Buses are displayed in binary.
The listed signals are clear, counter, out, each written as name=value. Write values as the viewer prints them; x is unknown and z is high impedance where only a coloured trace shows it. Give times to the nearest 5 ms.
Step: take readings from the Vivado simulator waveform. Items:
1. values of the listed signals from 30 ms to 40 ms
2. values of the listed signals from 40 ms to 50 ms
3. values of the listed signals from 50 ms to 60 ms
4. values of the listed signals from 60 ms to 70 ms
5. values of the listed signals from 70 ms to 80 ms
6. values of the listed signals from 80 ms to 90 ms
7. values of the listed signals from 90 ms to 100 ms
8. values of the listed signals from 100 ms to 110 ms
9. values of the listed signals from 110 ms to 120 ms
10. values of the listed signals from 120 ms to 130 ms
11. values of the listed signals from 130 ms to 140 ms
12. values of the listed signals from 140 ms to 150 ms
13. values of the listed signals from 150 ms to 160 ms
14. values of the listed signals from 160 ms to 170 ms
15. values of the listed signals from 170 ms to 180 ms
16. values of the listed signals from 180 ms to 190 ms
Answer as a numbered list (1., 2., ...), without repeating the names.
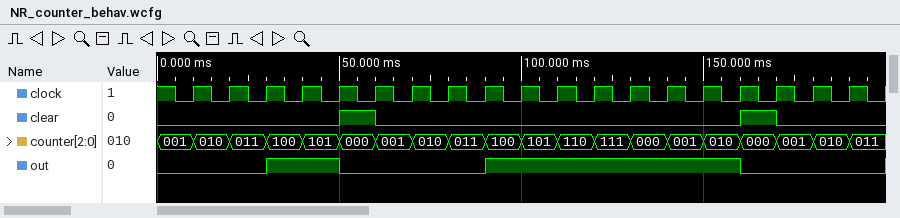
1. clear=0, counter=100, out=1
2. clear=0, counter=101, out=1
3. clear=1, counter=000, out=0
4. clear=0, counter=001, out=0
5. clear=0, counter=010, out=0
6. clear=0, counter=011, out=0
7. clear=0, counter=100, out=1
8. clear=0, counter=101, out=1
9. clear=0, counter=110, out=1
10. clear=0, counter=111, out=1
11. clear=0, counter=000, out=1
12. clear=0, counter=001, out=1
13. clear=0, counter=010, out=1
14. clear=1, counter=000, out=0
15. clear=0, counter=001, out=0
16. clear=0, counter=010, out=0
